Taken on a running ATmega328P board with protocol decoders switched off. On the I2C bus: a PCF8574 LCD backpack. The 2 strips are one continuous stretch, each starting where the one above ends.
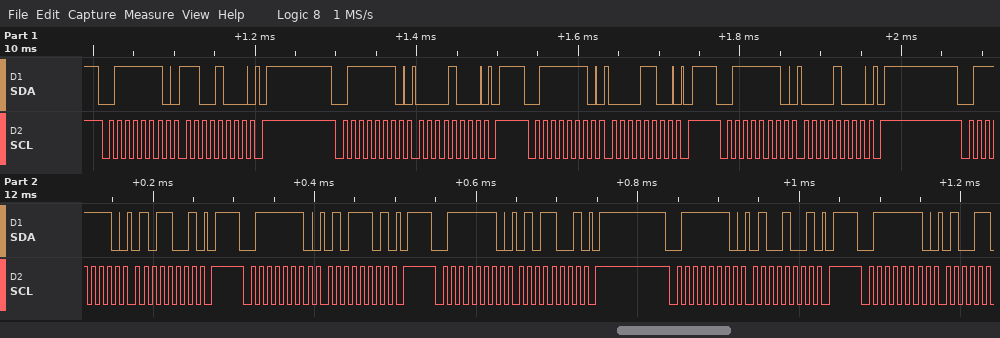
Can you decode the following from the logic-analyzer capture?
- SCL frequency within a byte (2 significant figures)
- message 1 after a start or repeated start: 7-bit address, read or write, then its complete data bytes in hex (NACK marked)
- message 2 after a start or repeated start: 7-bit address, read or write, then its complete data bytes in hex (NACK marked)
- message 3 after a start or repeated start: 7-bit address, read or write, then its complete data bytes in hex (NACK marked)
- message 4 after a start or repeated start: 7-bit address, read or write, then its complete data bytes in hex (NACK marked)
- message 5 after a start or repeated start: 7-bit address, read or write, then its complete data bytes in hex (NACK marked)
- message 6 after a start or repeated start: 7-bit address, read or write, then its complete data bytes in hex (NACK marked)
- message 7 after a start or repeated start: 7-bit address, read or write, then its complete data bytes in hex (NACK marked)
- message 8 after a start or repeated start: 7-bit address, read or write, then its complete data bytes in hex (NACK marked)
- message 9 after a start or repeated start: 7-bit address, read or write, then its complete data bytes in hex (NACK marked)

100 kHz
0x3F write: C8
0x3F write: 08
0x3F write: 0C
0x3F write: 08
0x3F write: 59
0x3F write: 5D
0x3F write: 59
0x3F write: 49
0x3F write
